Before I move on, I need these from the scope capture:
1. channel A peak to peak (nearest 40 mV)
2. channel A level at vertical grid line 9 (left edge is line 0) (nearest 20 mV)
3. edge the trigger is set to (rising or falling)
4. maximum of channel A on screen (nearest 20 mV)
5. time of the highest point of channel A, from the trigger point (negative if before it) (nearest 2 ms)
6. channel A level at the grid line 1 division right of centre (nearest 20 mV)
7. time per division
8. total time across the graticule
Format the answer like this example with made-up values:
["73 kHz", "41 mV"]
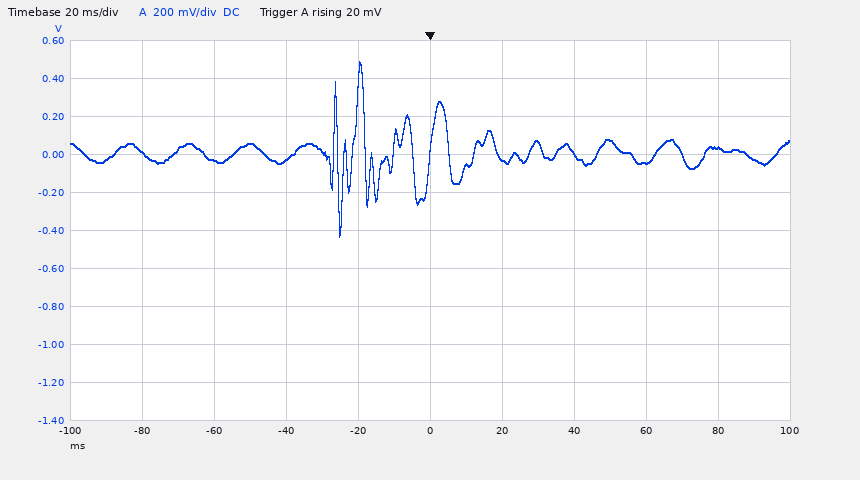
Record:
["920 mV", "40 mV", "rising", "480 mV", "-20 ms", "-20 mV", "20 ms", "200 ms"]
